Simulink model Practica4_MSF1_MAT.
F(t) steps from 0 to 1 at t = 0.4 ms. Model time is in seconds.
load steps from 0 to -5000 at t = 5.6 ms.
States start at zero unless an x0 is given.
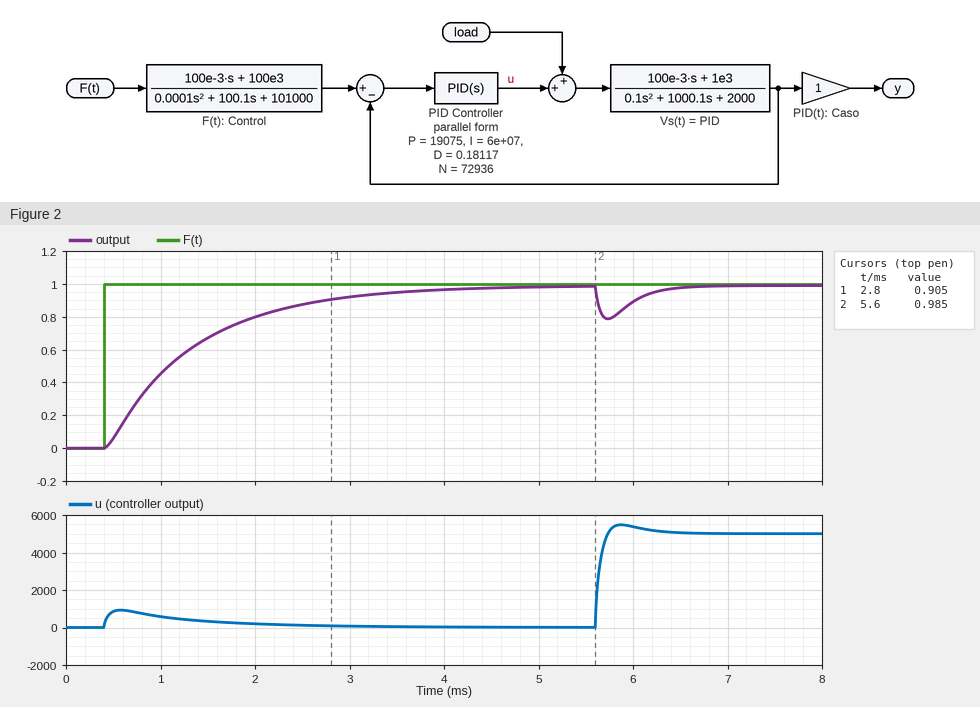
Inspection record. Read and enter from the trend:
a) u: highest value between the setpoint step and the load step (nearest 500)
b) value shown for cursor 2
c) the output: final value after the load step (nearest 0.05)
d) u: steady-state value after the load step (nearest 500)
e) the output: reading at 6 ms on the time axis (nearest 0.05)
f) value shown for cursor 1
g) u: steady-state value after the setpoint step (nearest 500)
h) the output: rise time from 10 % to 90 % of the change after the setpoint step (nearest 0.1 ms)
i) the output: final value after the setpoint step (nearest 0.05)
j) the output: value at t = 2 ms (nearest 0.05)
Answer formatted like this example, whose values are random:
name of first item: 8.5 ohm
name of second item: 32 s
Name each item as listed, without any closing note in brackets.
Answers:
u: highest value between the setpoint step and the load step: 1000
value shown for cursor 2: 0.985
the output: final value after the load step: 1.00
u: steady-state value after the load step: 5000
the output: reading at 6 ms on the time axis: 0.90
value shown for cursor 1: 0.905
u: steady-state value after the setpoint step: 0
the output: rise time from 10 % to 90 % of the change after the setpoint step: 2.1 ms
the output: final value after the setpoint step: 1.00
the output: value at t = 2 ms: 0.80
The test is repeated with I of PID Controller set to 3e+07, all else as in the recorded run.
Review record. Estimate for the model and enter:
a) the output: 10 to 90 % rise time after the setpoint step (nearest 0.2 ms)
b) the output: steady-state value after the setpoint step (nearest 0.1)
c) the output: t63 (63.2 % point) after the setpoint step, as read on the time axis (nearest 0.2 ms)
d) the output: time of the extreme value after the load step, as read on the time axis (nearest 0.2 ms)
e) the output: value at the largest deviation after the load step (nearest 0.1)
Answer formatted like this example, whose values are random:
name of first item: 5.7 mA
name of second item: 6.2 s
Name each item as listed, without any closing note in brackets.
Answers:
the output: 10 to 90 % rise time after the setpoint step: 2.0 ms
the output: steady-state value after the setpoint step: 1.0
the output: t63 (63.2 % point) after the setpoint step, as read on the time axis: 1.4 ms
the output: time of the extreme value after the load step, as read on the time axis: 5.8 ms
the output: value at the largest deviation after the load step: 0.8
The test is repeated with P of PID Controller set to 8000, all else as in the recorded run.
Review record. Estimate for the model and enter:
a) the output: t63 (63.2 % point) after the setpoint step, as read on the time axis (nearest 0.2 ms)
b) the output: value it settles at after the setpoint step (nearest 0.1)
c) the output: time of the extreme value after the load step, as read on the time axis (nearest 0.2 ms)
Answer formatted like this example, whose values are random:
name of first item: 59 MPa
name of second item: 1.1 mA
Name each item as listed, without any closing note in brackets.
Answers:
the output: t63 (63.2 % point) after the setpoint step, as read on the time axis: 1.4 ms
the output: value it settles at after the setpoint step: 1.0
the output: time of the extreme value after the load step, as read on the time axis: 5.8 ms
